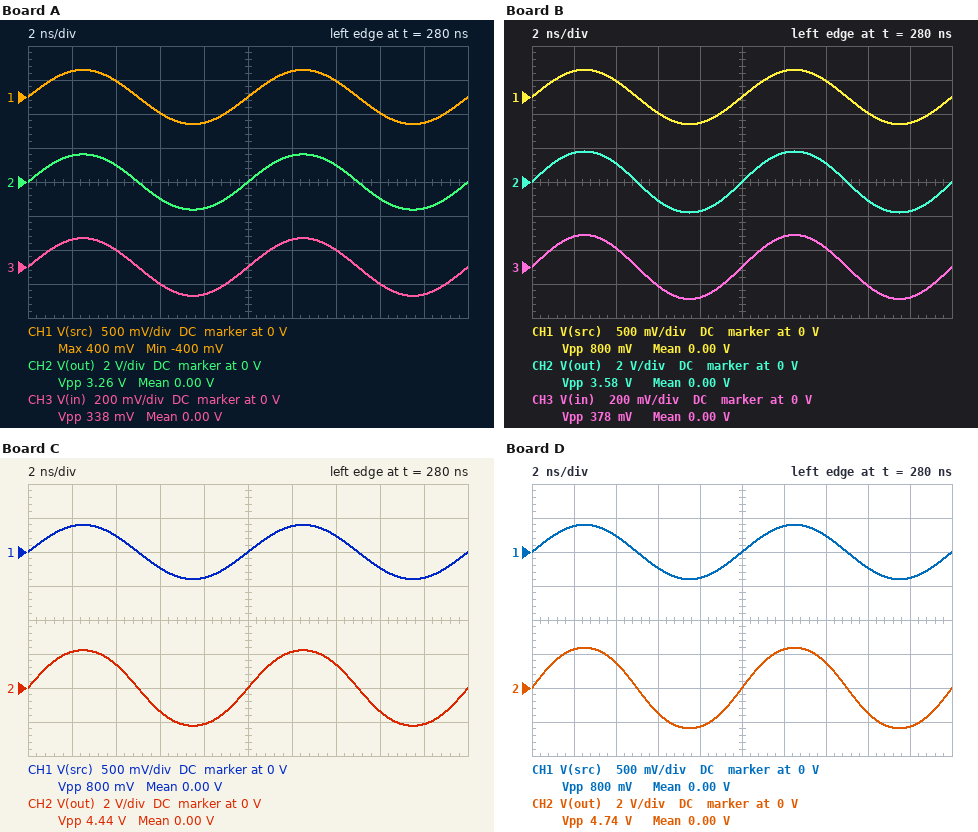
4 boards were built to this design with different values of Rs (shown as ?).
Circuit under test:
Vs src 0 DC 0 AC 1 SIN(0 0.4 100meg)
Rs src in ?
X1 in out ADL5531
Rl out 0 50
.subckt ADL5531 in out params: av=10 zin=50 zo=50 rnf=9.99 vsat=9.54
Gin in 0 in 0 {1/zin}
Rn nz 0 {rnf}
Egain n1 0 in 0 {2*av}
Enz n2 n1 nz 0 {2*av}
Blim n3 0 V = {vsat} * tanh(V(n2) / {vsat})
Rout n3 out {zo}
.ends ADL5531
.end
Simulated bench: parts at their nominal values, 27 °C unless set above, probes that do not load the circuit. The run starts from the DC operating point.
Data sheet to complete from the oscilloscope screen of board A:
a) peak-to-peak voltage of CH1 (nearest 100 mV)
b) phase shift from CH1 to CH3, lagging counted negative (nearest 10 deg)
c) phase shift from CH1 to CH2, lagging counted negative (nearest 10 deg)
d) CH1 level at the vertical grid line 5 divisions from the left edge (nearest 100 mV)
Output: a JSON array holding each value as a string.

["800 mV", "0 deg", "0 deg", "0 V"]
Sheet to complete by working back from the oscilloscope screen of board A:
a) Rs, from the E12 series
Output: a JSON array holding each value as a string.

["68 Ω"]
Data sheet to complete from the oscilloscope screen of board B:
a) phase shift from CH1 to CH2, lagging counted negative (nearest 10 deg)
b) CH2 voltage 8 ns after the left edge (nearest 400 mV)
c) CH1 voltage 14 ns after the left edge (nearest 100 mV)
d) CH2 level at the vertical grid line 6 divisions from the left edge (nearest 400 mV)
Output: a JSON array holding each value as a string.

["0 deg", "-1.6 V", "200 mV", "1.6 V"]
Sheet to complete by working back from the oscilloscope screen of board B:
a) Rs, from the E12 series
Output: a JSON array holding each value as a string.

["56 Ω"]
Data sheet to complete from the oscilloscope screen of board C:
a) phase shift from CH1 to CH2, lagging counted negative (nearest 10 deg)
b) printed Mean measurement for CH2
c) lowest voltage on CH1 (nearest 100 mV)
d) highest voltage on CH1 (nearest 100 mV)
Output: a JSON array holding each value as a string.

["0 deg", "0.00 V", "-400 mV", "400 mV"]
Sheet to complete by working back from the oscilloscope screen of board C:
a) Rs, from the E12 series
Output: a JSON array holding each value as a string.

["33 Ω"]
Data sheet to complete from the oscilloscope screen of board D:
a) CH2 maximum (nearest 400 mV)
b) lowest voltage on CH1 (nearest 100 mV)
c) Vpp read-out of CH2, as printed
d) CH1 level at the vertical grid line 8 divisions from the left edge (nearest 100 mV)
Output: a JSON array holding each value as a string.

["2.4 V", "-400 mV", "4.74 V", "-200 mV"]
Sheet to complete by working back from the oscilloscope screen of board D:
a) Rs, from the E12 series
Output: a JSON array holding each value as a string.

["27 Ω"]
